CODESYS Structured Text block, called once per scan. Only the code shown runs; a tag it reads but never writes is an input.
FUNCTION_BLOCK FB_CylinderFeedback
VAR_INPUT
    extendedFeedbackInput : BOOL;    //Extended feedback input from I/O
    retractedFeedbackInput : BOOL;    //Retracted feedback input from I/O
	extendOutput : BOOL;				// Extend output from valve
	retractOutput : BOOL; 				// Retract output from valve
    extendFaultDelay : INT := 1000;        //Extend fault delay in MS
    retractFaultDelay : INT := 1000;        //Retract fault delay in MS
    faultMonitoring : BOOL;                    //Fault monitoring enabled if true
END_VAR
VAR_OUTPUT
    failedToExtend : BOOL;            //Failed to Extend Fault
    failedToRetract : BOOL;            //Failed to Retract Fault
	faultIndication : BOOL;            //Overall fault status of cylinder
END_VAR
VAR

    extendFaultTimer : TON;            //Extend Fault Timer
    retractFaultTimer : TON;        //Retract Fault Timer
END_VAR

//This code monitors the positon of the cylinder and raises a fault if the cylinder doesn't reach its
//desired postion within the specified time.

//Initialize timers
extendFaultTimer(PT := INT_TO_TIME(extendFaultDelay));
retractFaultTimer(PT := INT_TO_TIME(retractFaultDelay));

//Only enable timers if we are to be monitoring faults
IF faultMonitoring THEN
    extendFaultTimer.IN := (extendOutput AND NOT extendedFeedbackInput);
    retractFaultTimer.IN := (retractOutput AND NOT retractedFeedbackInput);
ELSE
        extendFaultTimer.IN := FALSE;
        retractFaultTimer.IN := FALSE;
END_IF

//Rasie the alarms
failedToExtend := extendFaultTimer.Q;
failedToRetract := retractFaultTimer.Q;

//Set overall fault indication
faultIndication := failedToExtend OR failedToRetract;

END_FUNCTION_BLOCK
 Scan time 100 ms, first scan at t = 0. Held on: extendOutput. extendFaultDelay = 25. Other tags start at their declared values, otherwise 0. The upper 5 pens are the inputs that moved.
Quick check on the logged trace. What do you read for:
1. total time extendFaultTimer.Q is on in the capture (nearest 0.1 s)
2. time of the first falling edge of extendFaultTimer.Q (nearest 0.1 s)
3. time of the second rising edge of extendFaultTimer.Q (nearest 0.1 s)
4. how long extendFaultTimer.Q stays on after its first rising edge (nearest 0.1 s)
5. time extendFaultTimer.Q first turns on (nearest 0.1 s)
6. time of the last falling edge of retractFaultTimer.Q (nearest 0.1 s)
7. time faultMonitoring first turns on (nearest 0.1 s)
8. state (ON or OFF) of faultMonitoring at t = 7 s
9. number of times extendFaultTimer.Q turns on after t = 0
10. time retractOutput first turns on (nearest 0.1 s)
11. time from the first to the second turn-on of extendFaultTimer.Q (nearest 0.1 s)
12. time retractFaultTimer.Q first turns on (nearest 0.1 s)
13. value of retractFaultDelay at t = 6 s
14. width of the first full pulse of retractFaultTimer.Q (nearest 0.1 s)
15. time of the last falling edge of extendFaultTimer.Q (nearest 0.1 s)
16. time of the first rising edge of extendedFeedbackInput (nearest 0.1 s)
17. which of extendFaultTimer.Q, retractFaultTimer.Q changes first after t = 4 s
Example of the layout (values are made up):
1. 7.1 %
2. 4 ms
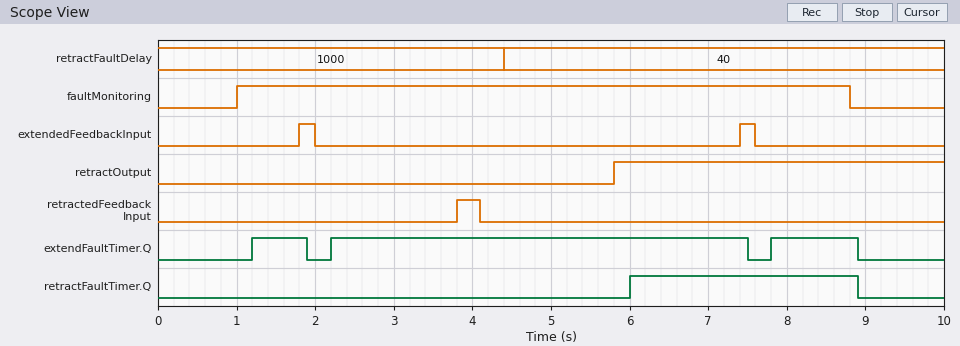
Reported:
1. 7.1 s
2. 1.9 s
3. 2.2 s
4. 0.7 s
5. 1.2 s
6. 8.9 s
7. 1.0 s
8. ON
9. 3
10. 5.8 s
11. 1.0 s
12. 6.0 s
13. 40
14. 2.9 s
15. 8.9 s
16. 1.8 s
17. retractFaultTimer.Q
